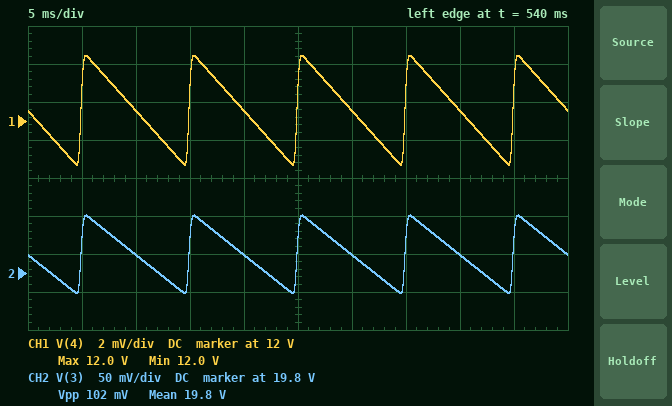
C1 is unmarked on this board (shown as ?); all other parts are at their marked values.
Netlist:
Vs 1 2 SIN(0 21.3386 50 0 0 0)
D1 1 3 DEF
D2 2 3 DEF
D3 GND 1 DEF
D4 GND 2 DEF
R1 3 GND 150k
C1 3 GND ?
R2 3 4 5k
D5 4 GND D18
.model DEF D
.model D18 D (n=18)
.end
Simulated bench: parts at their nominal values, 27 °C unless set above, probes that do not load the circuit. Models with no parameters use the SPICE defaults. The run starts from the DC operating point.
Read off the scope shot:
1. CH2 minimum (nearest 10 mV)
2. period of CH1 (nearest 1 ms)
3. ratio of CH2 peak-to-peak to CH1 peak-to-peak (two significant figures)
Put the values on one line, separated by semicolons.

19.77 V; 10 ms; 18
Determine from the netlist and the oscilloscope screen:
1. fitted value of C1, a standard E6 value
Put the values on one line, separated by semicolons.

150 µF
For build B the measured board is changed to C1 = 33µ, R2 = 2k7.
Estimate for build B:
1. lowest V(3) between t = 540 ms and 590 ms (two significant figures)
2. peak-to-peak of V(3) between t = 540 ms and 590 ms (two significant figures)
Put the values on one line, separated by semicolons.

19 V; 750 mV
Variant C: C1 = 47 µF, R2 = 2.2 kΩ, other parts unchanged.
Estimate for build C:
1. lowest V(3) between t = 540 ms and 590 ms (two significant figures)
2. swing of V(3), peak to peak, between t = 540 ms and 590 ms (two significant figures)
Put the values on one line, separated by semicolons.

19 V; 640 mV
